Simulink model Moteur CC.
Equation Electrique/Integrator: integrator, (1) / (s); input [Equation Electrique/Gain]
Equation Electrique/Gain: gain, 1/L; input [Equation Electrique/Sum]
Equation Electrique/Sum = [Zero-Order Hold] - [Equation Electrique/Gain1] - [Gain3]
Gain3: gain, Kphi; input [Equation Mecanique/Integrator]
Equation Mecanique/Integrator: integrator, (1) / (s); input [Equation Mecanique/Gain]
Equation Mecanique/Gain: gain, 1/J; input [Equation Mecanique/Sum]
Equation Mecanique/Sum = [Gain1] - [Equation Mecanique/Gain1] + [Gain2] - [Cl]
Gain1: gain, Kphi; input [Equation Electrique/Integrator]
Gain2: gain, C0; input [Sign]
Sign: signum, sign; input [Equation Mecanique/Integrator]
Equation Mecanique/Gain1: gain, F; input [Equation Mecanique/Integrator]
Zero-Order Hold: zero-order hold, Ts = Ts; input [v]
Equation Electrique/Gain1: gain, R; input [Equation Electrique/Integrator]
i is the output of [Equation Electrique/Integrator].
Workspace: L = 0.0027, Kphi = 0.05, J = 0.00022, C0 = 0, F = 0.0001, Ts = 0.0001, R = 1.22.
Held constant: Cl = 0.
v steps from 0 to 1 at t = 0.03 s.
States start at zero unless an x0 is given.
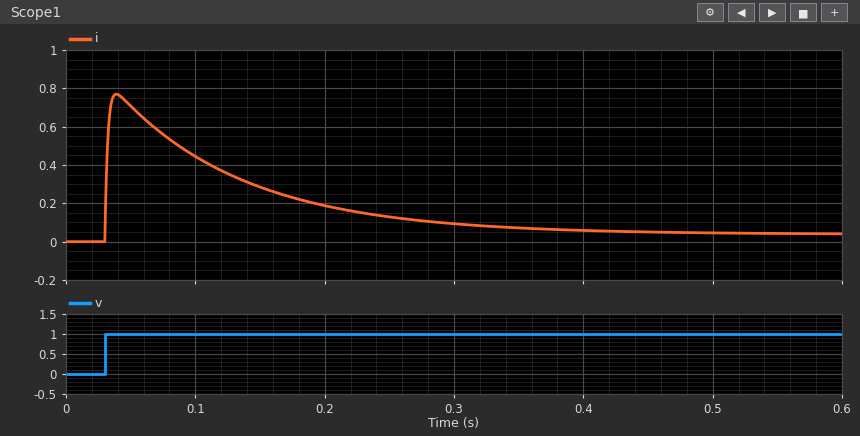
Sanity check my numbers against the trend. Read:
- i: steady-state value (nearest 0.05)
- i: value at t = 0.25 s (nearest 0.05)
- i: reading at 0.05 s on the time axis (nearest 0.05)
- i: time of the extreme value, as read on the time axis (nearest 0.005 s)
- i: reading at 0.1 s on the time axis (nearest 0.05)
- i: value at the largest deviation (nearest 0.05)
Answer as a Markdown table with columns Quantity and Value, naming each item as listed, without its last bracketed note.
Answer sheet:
| Quantity | Value |
|---|---|
| i: steady-state value | 0.05 |
| i: value at t = 0.25 s | 0.15 |
| i: reading at 0.05 s on the time axis | 0.70 |
| i: time of the extreme value, as read on the time axis | 0.040 s |
| i: reading at 0.1 s on the time axis | 0.45 |
| i: value at the largest deviation | 0.75 |
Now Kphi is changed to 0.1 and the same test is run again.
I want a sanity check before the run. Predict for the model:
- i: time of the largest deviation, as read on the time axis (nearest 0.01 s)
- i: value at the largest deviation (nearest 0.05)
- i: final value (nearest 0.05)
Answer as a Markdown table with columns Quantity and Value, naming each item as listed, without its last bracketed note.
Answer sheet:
| Quantity | Value |
|---|---|
| i: time of the largest deviation, as read on the time axis | 0.04 s |
| i: value at the largest deviation | 0.70 |
| i: final value | 0.00 |
